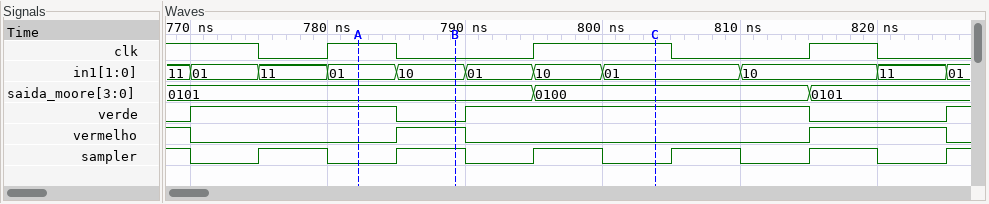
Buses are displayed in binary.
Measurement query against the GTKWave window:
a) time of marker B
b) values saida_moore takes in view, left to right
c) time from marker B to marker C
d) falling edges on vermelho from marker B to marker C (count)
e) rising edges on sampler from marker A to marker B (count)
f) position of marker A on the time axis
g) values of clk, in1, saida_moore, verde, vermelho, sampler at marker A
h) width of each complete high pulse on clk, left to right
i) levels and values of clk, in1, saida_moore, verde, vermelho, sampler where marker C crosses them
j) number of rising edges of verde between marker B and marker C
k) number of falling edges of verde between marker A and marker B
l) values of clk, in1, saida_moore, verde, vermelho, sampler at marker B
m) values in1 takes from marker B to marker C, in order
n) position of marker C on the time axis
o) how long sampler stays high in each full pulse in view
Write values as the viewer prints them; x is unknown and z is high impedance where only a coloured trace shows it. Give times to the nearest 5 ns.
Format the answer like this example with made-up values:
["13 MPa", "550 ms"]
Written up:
["790 ns", "0101, 0100, 0101", "15 ns", "1", "1", "780 ns", "clk=1, in1=01, saida_moore=0101, verde=1, vermelho=0, sampler=0", "5 ns, 10 ns, 5 ns", "clk=1, in1=01, saida_moore=0100, verde=1, vermelho=0, sampler=0", "1", "1", "clk=0, in1=10, saida_moore=0101, verde=0, vermelho=1, sampler=1", "10, 01, 10, 01", "805 ns", "5 ns, 5 ns, 5 ns, 5 ns, 5 ns"]
